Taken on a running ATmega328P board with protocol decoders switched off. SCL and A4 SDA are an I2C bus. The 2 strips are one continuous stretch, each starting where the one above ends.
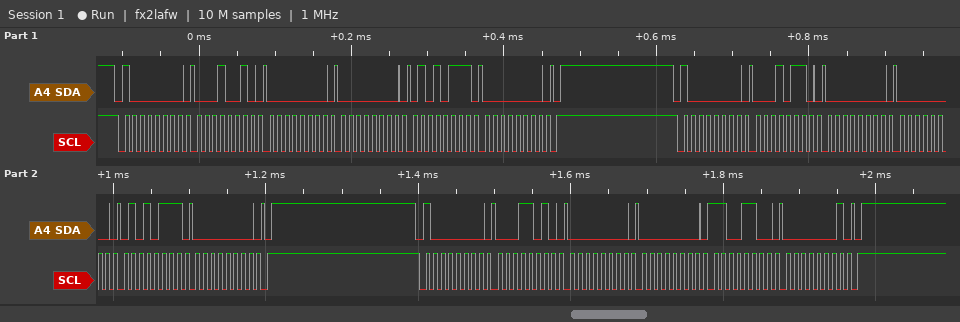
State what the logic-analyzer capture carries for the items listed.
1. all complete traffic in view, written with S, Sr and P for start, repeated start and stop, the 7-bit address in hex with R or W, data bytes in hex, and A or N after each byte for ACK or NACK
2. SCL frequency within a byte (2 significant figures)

S 40W A 12 A 00 A 00 A 57 A 00 A P S 40W A 16 A 00 A 00 A 57 A 00 A P S 40W A 1A A 00 A 00 A CC A 01 A P
100 kHz
